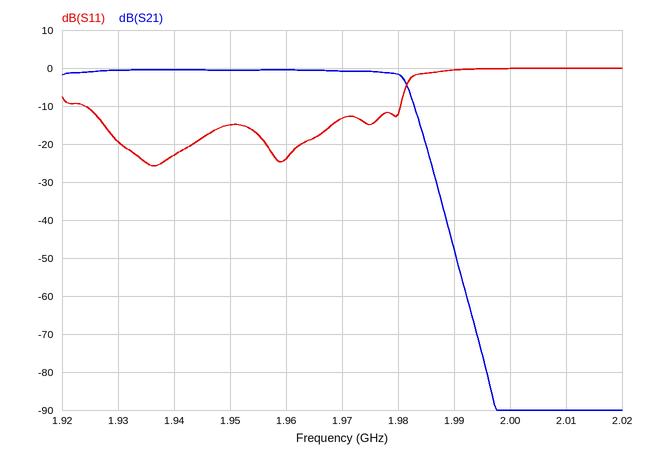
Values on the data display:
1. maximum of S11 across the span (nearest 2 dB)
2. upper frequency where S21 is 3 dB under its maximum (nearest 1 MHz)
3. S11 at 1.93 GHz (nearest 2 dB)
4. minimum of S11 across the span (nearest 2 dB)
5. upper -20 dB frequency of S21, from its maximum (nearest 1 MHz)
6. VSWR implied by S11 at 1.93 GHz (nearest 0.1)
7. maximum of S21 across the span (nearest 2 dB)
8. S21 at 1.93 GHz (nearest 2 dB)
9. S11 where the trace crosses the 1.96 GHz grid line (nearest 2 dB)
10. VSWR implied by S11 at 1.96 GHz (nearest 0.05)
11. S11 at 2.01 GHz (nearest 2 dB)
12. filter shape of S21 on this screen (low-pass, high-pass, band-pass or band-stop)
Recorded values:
0 dB
1.981 GHz
-20 dB
-26 dB
1.985 GHz
1.2
0 dB
0 dB
-24 dB
1.15
0 dB
low-pass
